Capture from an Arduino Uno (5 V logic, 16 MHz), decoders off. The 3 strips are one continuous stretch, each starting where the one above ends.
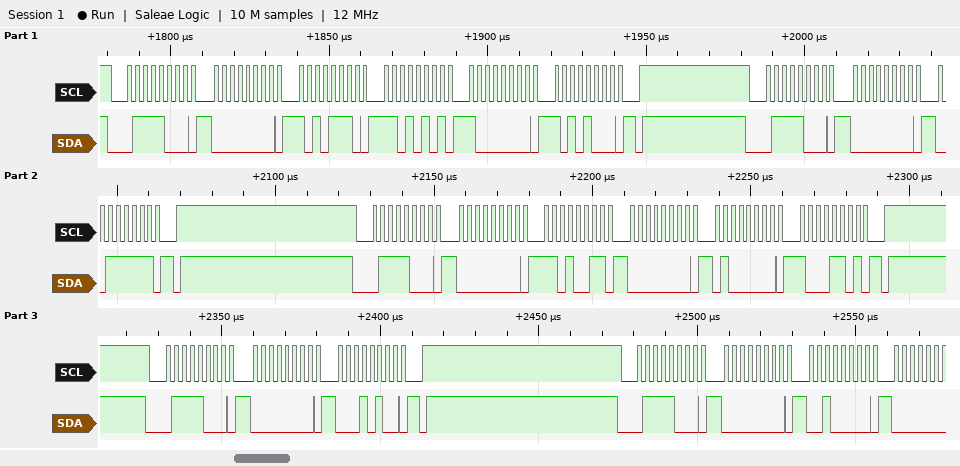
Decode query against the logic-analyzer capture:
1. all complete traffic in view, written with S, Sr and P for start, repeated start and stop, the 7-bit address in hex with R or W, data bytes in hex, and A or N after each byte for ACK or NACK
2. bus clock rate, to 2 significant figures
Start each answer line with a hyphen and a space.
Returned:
- S 3CW A 00 A AE A D5 A 80 A A8 A P S 3CW A 00 A 3F A P S 3CW A 00 A D3 A 00 A 40 A 8D A P S 3CW A 00 A 14 A P S 3CW A 00 A 20 A
- 400 kHz
